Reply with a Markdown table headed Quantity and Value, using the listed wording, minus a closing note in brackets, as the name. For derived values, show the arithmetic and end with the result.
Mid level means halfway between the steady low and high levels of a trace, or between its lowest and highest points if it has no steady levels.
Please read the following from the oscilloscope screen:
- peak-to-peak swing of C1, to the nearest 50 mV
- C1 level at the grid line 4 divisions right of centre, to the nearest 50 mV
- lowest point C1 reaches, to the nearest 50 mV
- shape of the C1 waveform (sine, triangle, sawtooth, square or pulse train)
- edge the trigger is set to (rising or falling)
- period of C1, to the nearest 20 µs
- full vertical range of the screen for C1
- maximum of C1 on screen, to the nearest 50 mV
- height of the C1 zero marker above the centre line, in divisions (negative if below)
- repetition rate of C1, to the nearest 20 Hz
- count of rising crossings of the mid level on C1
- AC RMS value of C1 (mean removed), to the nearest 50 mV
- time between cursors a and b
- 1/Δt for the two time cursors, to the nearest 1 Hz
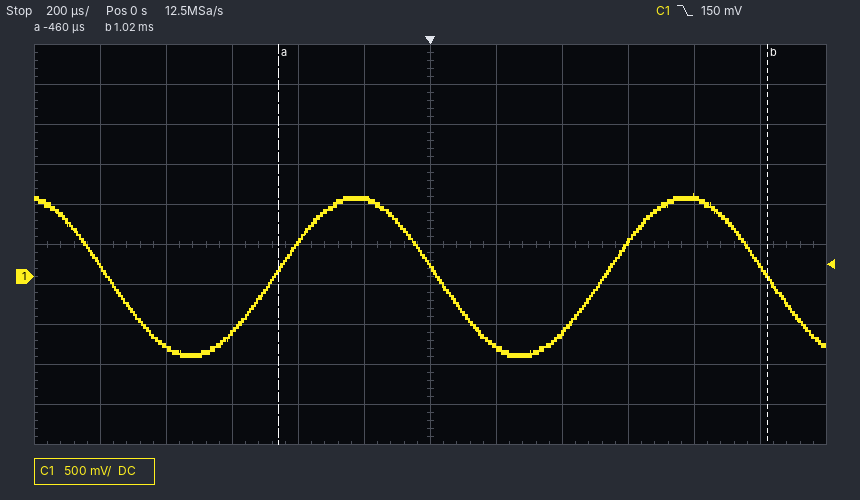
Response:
| Quantity | Value |
|---|---|
| peak-to-peak swing of C1, to the nearest 50 mV | 1.05 V − (-1.00 V) = 2.05 V |
| C1 level at the grid line 4 divisions right of centre, to the nearest 50 mV | 1.00 V |
| lowest point C1 reaches, to the nearest 50 mV | -1.00 V |
| shape of the C1 waveform | sine |
| edge the trigger is set to | falling |
| period of C1, to the nearest 20 µs | 1.00 ms |
| full vertical range of the screen for C1 | 5 V |
| maximum of C1 on screen, to the nearest 50 mV | 1.05 V |
| height of the C1 zero marker above the centre line, in divisions | -0.8 div |
| repetition rate of C1, to the nearest 20 Hz | 1 / 1.00 ms ≈ 1.00 kHz |
| count of rising crossings of the mid level on C1 | 2 |
| AC RMS value of C1 (mean removed), to the nearest 50 mV | 2.05 V / (2√2) ≈ 725 mV, so 700 mV to the nearest 50 mV |
| time between cursors a and b | 1.02 ms − (-460 µs) = 1.48 ms |
| 1/Δt for the two time cursors, to the nearest 1 Hz | 1 / 1.48 ms ≈ 676 Hz |
